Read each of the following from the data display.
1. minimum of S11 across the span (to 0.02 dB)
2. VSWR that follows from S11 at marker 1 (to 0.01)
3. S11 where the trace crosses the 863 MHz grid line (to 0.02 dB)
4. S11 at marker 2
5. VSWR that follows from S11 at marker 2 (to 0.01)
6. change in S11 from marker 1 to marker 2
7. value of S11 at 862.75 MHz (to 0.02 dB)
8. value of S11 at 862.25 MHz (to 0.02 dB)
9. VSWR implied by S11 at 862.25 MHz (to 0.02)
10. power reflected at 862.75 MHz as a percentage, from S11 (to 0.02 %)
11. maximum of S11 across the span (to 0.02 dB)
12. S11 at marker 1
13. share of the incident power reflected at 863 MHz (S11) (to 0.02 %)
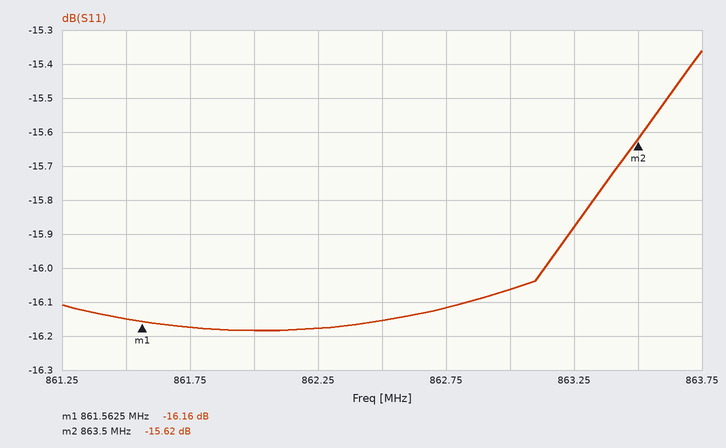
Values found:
-16.18 dB
1.37
-16.06 dB
-15.62 dB
1.40
0.54 dB
-16.12 dB
-16.18 dB
1.36
2.44 %
-15.36 dB
-16.16 dB
2.48 %
